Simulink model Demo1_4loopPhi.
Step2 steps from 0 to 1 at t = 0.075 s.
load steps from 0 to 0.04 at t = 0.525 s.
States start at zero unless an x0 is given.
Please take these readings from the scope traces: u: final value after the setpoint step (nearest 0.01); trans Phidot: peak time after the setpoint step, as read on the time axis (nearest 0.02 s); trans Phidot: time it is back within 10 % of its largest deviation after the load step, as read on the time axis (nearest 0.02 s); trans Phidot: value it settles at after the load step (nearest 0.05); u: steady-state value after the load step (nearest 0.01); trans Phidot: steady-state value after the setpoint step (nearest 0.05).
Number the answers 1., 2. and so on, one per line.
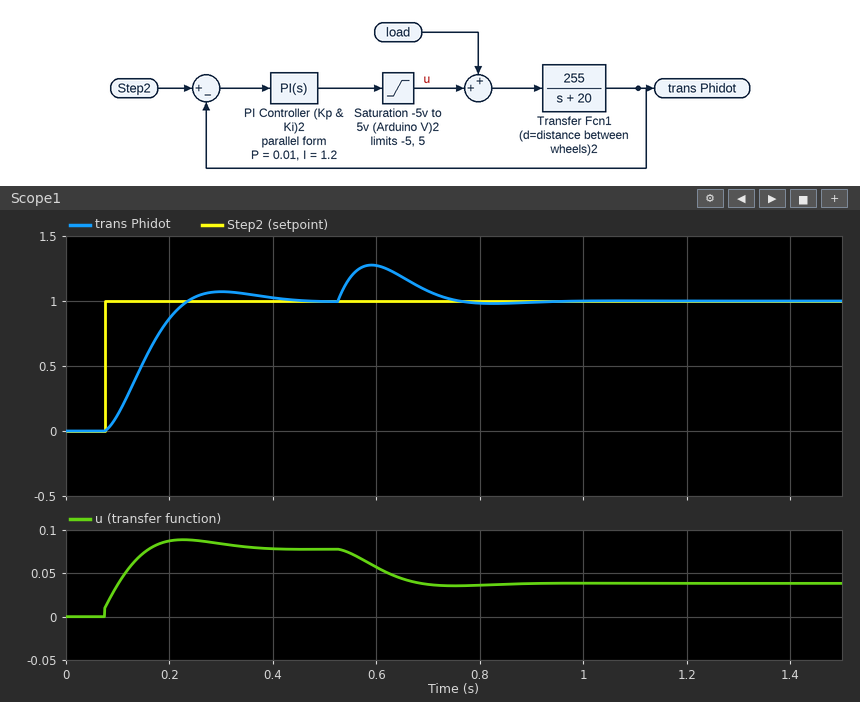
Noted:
1. 0.08
2. 0.30 s
3. 0.74 s
4. 1.00
5. 0.04
6. 1.00
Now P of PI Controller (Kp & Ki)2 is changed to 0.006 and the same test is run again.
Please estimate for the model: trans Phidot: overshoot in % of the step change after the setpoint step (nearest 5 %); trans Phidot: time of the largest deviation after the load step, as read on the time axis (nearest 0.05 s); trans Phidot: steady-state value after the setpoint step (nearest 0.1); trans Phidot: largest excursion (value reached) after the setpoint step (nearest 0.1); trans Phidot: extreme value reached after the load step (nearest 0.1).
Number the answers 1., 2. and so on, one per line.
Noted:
1. 10 %
2. 0.60 s
3. 1.0
4. 1.1
5. 1.3
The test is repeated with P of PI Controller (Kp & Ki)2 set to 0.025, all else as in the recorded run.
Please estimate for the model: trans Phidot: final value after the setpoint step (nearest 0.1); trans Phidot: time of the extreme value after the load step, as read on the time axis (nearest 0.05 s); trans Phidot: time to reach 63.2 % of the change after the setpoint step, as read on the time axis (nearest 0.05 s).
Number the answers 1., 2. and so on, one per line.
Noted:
1. 1.0
2. 0.60 s
3. 0.15 s
